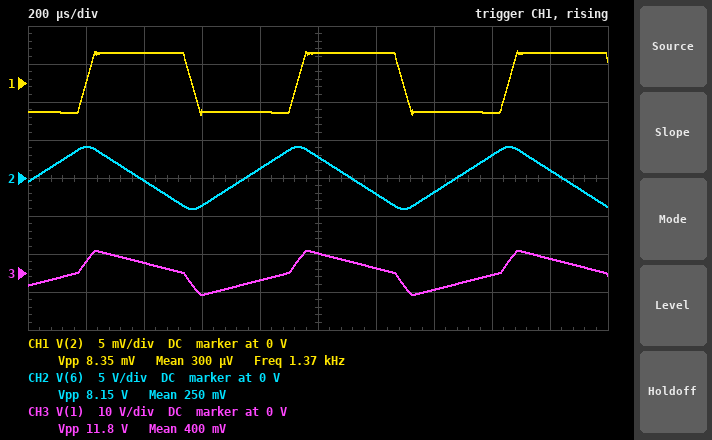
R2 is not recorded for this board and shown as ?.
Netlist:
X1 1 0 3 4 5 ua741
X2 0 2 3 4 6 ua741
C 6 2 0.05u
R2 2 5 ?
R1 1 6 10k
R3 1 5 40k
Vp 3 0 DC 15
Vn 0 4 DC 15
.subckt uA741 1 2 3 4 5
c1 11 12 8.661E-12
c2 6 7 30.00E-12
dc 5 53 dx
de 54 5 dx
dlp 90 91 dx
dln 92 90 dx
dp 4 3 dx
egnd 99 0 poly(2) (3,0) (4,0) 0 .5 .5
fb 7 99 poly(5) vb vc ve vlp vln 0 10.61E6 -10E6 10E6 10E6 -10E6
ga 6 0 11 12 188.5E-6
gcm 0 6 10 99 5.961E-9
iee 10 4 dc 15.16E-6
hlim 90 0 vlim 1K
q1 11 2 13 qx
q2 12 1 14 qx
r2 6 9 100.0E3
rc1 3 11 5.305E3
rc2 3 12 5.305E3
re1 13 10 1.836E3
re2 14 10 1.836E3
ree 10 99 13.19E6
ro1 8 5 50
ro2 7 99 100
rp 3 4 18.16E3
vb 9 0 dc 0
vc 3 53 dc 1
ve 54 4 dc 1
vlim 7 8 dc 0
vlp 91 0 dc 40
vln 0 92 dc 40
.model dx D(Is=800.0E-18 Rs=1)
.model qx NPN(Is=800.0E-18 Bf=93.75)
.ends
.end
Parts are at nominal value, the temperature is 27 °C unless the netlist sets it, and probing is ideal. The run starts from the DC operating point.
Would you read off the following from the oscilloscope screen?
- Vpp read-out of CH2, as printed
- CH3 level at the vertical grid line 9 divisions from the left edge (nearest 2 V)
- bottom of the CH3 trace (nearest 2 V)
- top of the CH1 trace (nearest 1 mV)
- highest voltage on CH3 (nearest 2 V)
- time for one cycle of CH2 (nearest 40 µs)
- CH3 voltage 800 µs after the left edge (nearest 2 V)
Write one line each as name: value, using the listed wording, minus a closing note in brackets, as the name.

Vpp read-out of CH2, as printed: 8.15 V
CH3 level at the vertical grid line 9 divisions from the left edge: 4 V
bottom of the CH3 trace: -6 V
top of the CH1 trace: 4 mV
highest voltage on CH3: 6 V
time for one cycle of CH2: 720 µs
CH3 voltage 800 µs after the left edge: -2 V
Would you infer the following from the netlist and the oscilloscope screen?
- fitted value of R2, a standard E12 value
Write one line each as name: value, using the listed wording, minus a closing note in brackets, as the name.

fitted value of R2, a standard E12 value: 12 kΩ
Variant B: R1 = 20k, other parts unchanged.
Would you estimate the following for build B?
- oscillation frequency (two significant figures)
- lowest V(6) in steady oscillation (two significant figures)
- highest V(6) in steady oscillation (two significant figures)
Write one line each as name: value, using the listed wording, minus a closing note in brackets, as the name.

oscillation frequency: 750 Hz
lowest V(6) in steady oscillation: -7.7 V
highest V(6) in steady oscillation: 7.7 V
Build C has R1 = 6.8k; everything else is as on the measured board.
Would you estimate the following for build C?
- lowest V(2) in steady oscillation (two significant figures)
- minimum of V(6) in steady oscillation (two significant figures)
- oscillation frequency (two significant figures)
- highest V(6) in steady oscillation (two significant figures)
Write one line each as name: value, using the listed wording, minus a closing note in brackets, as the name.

lowest V(2) in steady oscillation: -4.2 mV
minimum of V(6) in steady oscillation: -2.9 V
oscillation frequency: 1.9 kHz
highest V(6) in steady oscillation: 2.9 V
